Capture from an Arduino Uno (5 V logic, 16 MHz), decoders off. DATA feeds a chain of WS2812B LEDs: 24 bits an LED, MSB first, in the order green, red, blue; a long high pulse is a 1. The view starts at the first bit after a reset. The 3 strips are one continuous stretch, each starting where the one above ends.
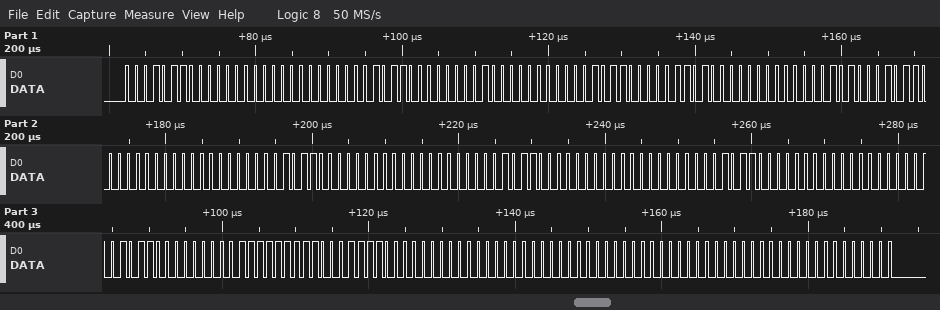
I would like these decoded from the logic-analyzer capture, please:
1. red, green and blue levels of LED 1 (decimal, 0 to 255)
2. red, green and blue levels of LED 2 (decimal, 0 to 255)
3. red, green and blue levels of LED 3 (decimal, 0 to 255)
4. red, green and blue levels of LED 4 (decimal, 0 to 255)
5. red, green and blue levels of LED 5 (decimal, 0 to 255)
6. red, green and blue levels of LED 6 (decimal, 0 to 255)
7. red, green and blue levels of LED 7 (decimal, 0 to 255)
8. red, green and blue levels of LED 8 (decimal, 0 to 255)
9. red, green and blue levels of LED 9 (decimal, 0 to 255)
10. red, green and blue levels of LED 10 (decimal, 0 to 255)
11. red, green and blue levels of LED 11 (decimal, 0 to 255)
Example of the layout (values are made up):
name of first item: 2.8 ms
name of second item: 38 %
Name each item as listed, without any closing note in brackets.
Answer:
red, green and blue levels of LED 1: 0, 22, 0
red, green and blue levels of LED 2: 1, 22, 0
red, green and blue levels of LED 3: 13, 22, 0
red, green and blue levels of LED 4: 22, 5, 0
red, green and blue levels of LED 5: 22, 0, 0
red, green and blue levels of LED 6: 22, 0, 0
red, green and blue levels of LED 7: 22, 0, 0
red, green and blue levels of LED 8: 22, 0, 0
red, green and blue levels of LED 9: 143, 255, 0
red, green and blue levels of LED 10: 0, 0, 0
red, green and blue levels of LED 11: 0, 0, 0
